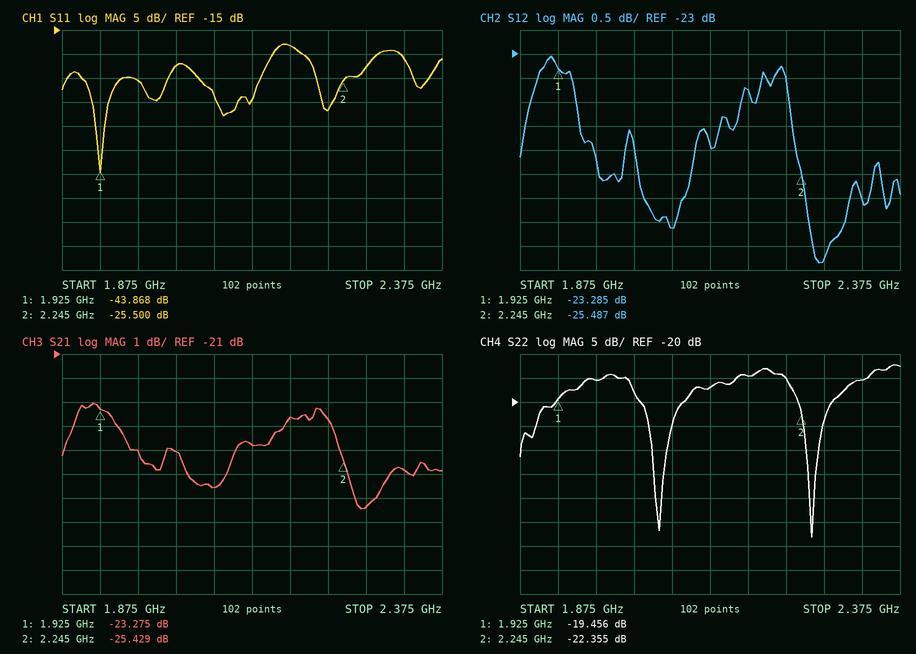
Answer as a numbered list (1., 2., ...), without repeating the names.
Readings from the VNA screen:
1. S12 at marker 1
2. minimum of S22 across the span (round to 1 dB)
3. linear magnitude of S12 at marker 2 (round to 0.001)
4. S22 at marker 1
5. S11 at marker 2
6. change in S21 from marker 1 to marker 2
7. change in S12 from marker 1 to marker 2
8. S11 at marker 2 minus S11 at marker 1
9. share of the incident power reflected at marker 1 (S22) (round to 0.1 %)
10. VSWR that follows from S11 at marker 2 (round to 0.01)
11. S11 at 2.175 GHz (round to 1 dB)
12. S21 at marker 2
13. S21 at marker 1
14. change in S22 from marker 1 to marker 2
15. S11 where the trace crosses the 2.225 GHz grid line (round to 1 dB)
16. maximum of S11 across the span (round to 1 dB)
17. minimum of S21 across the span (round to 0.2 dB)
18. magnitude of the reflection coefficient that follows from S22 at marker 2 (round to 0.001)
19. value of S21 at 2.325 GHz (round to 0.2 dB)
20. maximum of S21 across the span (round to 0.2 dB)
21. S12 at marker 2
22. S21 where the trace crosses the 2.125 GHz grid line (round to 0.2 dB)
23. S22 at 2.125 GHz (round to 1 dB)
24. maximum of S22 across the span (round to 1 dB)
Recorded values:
1. -23.285 dB
2. -48 dB
3. 0.053
4. -19.456 dB
5. -25.500 dB
6. -2.154 dB
7. -2.202 dB
8. 18.368 dB
9. 1.1 %
10. 1.11
11. -18 dB
12. -25.429 dB
13. -23.275 dB
14. -2.899 dB
15. -32 dB
16. -18 dB
17. -27.4 dB
18. 0.076
19. -25.8 dB
20. -23.0 dB
21. -25.487 dB
22. -24.8 dB
23. -17 dB
24. -12 dB
